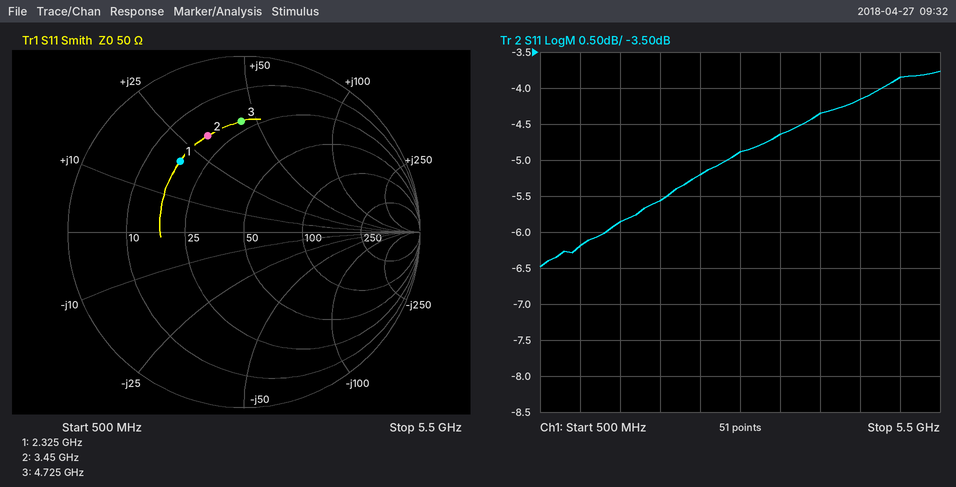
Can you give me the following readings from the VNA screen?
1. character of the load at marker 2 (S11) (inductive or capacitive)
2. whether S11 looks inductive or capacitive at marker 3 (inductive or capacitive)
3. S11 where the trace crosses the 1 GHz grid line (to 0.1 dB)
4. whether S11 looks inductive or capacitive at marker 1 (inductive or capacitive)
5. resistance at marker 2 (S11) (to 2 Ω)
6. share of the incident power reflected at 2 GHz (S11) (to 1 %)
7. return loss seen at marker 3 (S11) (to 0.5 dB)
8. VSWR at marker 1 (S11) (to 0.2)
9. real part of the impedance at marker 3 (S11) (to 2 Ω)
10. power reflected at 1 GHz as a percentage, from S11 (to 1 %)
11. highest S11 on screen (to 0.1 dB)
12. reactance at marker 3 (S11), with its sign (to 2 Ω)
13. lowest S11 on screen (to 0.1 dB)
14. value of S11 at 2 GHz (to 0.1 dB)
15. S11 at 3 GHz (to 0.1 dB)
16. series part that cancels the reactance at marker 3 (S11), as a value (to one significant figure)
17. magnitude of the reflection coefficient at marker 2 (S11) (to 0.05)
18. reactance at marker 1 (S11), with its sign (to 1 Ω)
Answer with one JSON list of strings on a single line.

["inductive", "inductive", "-6.2 dB", "inductive", "18 Ω", "28 %", "4.0 dB", "3.4", "22 Ω", "24 %", "-3.8 dB", "+44 Ω", "-6.5 dB", "-5.6 dB", "-4.9 dB", "800 fF", "0.60", "+20 Ω"]
